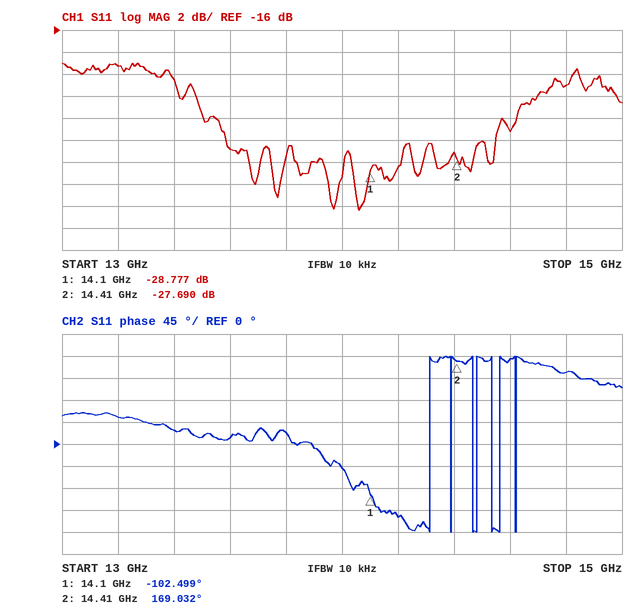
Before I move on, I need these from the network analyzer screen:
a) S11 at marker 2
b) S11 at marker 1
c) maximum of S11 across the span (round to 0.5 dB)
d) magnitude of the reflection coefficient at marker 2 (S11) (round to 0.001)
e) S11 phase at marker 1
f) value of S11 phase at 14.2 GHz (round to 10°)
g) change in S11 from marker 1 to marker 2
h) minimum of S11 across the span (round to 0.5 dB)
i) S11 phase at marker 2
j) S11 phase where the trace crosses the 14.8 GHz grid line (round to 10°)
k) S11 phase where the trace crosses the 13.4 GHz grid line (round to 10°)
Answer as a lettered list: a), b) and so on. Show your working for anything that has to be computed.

a) -27.690 dB
b) -28.777 dB
c) -19.0 dB
d) 10^(-27.69/20) ≈ 0.041
e) -102.499°
f) -150°
g) -27.69 − (-28.777) = 1.087 dB
h) -32.5 dB
i) 169.032°
j) 150°
k) 30°
